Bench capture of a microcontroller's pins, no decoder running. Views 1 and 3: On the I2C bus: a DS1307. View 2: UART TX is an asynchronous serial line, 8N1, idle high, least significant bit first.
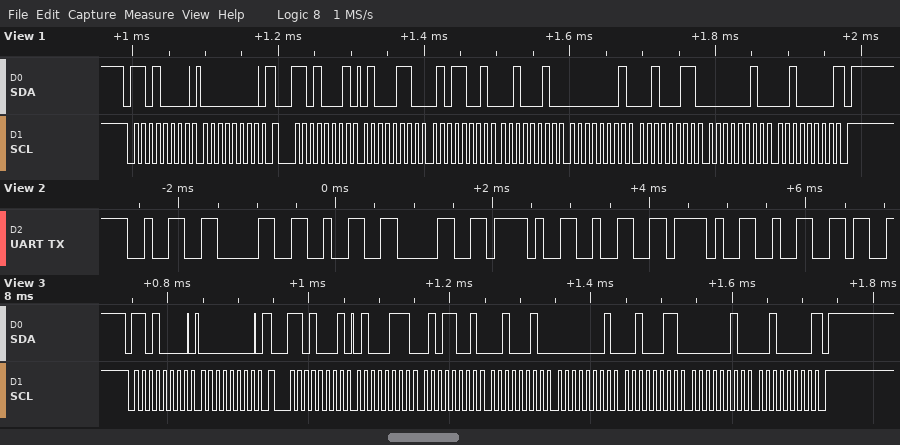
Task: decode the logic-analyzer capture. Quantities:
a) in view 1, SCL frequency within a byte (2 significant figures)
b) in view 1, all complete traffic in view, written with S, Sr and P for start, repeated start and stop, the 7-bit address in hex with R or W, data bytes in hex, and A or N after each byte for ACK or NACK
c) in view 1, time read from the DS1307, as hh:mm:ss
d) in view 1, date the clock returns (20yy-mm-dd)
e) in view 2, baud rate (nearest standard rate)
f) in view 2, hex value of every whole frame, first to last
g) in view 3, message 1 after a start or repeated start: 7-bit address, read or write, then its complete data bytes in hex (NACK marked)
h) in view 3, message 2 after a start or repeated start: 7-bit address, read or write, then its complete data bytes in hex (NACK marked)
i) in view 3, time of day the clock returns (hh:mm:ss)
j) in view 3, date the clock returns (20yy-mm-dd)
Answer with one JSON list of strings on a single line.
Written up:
["100 kHz", "S 68W A 00 A Sr 68R A 46 A 59 A 22 A 01 A 23 A 02 A 20 N P", "22:59:46", "2020-02-23", "9600 baud", "0x32 0x30 0x32 0x30 0x2F 0x32 0x2F 0x32", "0x68 write: 00", "0x68 read: 47 59 22 01 23 02 20 NACK", "22:59:47", "2020-02-23"]
